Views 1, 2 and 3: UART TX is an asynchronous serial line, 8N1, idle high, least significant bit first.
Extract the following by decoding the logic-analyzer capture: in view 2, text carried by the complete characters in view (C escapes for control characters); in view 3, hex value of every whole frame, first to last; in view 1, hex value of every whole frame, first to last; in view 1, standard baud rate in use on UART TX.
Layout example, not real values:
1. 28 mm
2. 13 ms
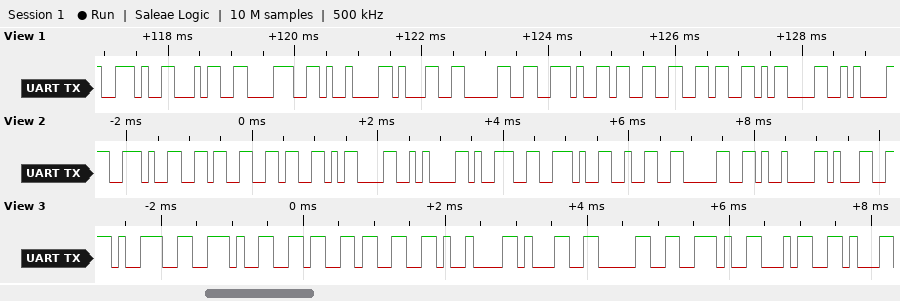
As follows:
1. ".66\r\n9.20\t1"
2. 39 2E 36 33 09 31 30 2E 34
3. 2E 34 38 09 31 30 2E 33 36 0D 0A
4. 9600 baud
